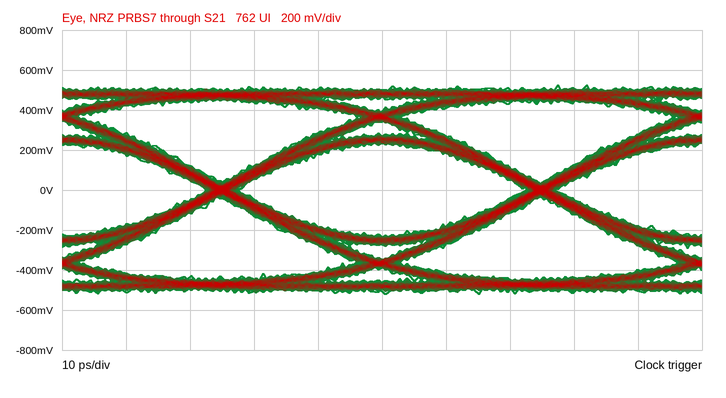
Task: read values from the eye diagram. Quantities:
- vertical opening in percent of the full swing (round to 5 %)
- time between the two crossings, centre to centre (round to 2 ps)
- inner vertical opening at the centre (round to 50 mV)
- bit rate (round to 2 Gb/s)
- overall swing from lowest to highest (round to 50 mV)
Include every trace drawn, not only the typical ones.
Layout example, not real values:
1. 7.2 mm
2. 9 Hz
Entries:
1. 45 %
2. 50 ps
3. 450 mV
4. 20 Gb/s
5. 1.05 V
